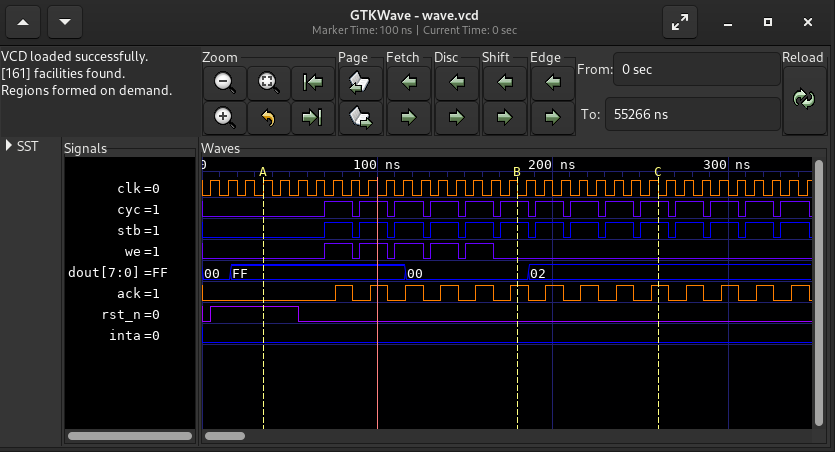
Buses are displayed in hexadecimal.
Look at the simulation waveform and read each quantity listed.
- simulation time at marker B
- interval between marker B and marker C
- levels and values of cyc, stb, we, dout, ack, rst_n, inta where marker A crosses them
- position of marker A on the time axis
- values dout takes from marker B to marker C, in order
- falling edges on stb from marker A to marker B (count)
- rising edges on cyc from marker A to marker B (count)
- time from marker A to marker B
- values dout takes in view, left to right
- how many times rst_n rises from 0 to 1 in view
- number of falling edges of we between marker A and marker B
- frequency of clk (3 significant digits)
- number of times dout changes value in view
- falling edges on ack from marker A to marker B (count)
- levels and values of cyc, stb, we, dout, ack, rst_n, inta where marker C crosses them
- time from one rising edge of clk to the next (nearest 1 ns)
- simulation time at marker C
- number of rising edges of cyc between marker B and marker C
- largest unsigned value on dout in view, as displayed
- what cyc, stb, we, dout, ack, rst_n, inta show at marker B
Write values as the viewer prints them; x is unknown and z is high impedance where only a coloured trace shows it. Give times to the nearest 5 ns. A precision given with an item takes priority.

180 ns
80 ns
cyc=0, stb=0, we=0, dout=FF, ack=0, rst_n=1, inta=0
35 ns
00, 02
5
6
145 ns
00, FF, 00, 02
1
5
100 MHz
3
5
cyc=1, stb=1, we=0, dout=02, ack=1, rst_n=0, inta=0
10 ns
260 ns
4
FF
cyc=1, stb=1, we=0, dout=00, ack=1, rst_n=0, inta=0
